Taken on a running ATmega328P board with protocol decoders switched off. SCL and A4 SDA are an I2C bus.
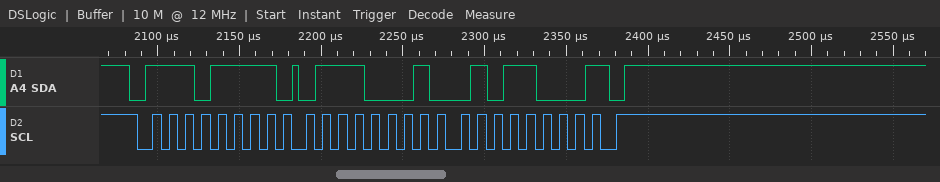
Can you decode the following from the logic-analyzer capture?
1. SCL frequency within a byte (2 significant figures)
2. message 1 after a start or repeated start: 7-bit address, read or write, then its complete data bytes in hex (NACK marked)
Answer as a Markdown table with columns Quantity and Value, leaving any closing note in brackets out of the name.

| Quantity | Value |
|---|---|
| SCL frequency within a byte | 100 kHz |
| message 1 after a start or repeated start: 7-bit address, read or write, then its complete data bytes in hex | 0x77 read: 71 58 NACK |
